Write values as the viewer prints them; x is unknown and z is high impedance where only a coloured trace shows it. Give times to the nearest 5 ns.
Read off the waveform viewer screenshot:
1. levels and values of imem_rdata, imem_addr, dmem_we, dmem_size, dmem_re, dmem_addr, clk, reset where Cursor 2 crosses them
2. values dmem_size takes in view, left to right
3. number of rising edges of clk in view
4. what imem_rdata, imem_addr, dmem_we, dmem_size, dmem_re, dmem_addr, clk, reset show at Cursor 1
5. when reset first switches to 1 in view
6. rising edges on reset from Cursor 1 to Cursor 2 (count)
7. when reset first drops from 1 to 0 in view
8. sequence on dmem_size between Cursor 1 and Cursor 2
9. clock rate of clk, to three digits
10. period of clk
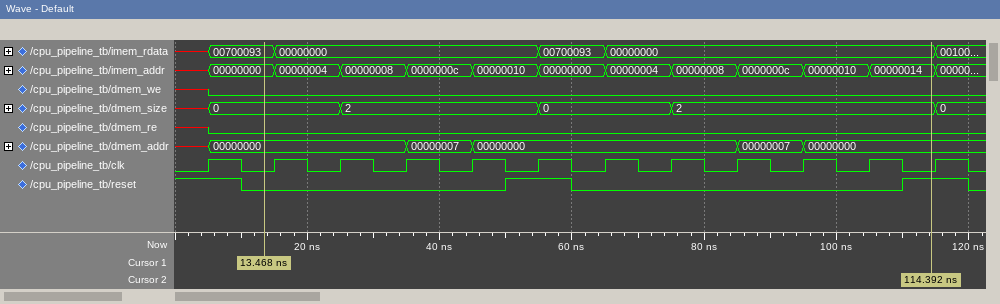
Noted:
imem_rdata=00000000, imem_addr=00000014, dmem_we=0, dmem_size=2, dmem_re=0, dmem_addr=00000000, clk=0, reset=1
x, 0, 2, 0, 2, 0
12
imem_rdata=00700093, imem_addr=00000000, dmem_we=0, dmem_size=0, dmem_re=0, dmem_addr=00000000, clk=0, reset=0
50 ns
2
10 ns
0, 2, 0, 2
100 MHz
10 ns
